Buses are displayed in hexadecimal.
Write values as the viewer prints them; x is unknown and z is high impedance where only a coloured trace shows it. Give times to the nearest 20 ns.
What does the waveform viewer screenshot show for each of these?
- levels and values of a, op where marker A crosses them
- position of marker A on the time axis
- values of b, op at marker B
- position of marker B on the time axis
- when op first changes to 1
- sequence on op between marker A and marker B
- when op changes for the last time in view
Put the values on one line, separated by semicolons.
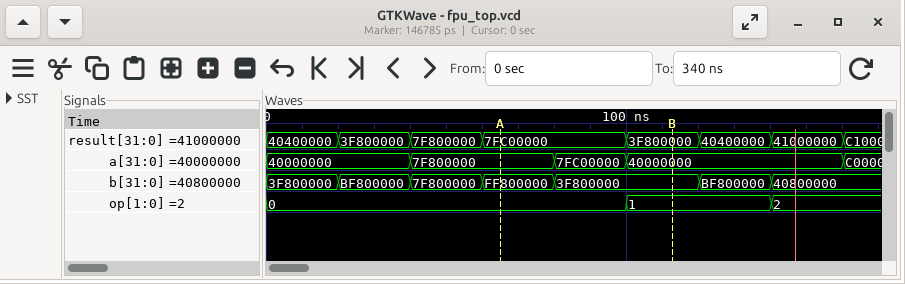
a=7F800000, op=0; 60 ns; b=3F800000, op=1; 120 ns; 100 ns; 0, 1; 140 ns
